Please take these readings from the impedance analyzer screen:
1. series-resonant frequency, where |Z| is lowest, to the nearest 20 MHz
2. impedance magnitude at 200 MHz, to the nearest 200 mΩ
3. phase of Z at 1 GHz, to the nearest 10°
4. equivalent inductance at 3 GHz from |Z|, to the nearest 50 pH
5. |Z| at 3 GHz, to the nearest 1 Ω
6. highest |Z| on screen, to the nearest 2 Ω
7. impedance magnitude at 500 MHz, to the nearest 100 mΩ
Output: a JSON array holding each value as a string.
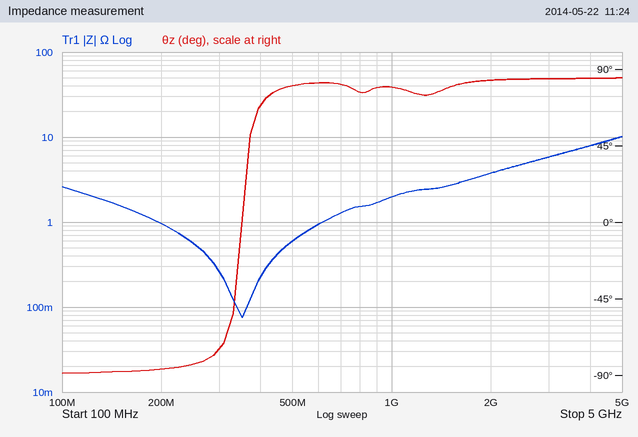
["360 MHz", "1.0 Ω", "80°", "300 pH", "6 Ω", "10 Ω", "600 mΩ"]
